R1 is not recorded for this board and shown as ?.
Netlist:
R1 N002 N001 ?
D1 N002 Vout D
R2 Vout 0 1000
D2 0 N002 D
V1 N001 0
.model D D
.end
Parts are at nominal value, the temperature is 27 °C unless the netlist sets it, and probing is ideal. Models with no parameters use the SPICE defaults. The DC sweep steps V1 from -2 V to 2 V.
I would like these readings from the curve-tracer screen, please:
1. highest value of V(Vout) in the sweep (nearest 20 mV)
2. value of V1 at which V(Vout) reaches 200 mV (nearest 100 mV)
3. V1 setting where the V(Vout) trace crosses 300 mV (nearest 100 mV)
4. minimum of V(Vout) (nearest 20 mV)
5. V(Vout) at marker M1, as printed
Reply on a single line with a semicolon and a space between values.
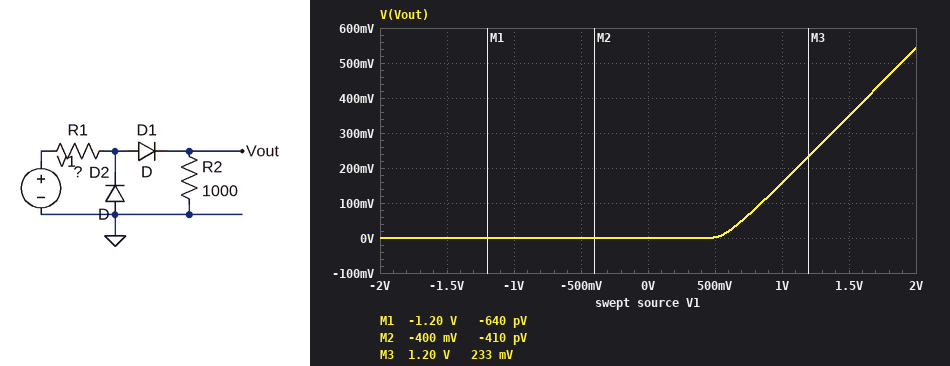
540 mV; 1.1 V; 1.4 V; 0 V; -640 pV
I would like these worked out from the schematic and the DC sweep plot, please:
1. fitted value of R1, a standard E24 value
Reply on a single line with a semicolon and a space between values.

1.5 kΩ
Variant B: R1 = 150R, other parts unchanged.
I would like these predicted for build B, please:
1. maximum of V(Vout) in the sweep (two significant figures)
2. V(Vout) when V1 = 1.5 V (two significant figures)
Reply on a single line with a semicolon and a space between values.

1.2 V; 740 mV
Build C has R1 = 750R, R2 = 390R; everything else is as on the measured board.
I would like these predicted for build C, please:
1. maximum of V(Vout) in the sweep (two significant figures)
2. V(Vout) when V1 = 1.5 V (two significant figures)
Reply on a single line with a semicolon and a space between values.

460 mV; 290 mV
